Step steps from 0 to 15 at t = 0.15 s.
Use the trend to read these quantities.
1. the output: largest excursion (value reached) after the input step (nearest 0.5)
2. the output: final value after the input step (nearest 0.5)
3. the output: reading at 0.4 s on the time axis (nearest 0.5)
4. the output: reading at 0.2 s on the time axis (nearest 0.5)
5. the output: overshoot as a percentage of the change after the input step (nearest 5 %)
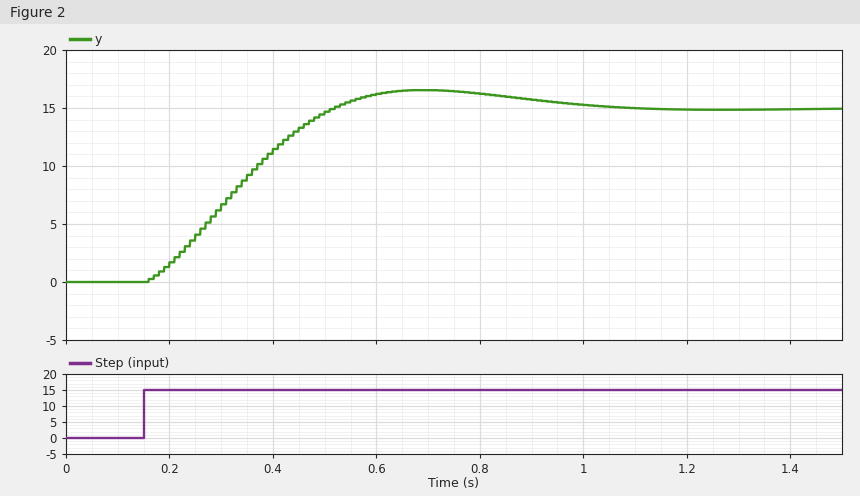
16.5
15.0
11.5
1.5
10 %
